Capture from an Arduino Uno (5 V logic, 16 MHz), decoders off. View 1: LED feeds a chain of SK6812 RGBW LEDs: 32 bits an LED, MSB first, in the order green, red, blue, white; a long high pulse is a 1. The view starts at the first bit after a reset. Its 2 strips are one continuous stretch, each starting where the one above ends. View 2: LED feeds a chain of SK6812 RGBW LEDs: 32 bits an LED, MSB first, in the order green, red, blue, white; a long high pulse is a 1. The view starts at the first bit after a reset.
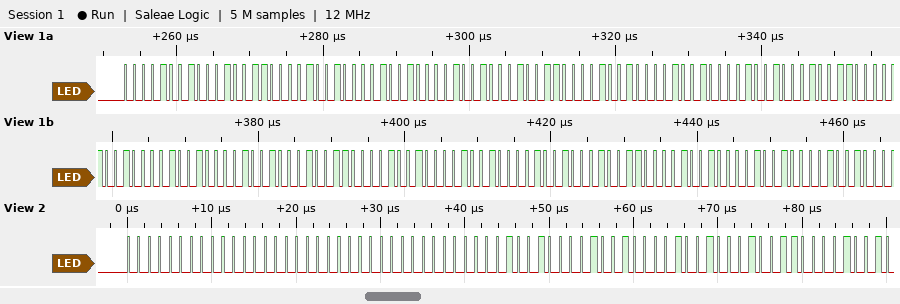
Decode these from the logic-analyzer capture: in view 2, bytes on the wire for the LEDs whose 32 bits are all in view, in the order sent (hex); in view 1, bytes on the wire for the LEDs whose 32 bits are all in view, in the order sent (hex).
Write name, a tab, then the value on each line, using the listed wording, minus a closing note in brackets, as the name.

in view 2, bytes on the wire for the LEDs whose 32 bits are all in view, in the order sent	00 00 00 00 09 09 09 13
in view 1, bytes on the wire for the LEDs whose 32 bits are all in view, in the order sent	09 13 09 09 09 13 09 09 09 13 09 09 09 13 09 09 09 13 09 09
